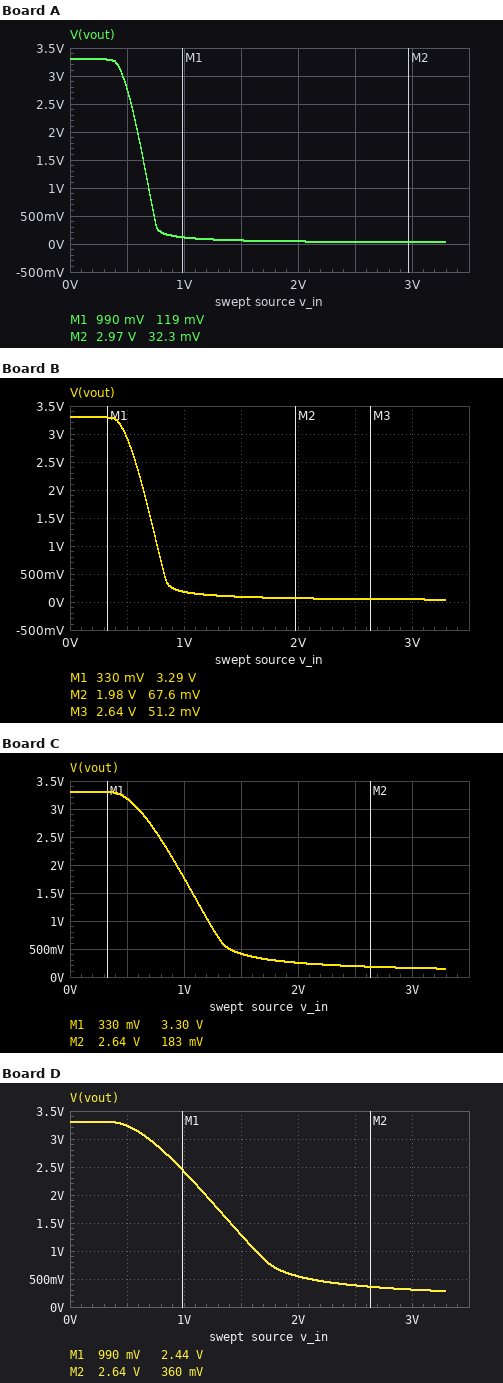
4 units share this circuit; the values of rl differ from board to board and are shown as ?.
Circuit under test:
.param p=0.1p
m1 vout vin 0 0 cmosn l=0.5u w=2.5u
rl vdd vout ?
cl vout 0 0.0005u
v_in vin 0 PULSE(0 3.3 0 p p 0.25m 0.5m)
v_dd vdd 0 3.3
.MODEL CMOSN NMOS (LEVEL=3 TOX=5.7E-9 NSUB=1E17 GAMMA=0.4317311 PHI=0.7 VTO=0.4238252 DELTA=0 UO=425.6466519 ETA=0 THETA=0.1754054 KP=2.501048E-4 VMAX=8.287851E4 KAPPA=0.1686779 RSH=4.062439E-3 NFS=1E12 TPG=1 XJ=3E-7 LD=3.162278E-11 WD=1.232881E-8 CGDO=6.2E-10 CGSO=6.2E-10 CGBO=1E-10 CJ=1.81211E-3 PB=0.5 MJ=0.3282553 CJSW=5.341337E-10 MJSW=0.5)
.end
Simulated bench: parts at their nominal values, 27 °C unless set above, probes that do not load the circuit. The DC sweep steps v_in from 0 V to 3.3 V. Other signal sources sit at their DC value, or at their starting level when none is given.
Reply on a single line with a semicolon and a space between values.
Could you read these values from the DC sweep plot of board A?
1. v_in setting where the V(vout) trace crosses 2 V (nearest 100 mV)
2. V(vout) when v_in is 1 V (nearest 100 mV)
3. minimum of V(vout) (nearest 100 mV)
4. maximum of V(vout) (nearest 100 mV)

600 mV; 100 mV; 0 V; 3.3 V
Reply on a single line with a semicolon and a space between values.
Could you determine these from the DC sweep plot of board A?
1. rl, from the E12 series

47 kΩ
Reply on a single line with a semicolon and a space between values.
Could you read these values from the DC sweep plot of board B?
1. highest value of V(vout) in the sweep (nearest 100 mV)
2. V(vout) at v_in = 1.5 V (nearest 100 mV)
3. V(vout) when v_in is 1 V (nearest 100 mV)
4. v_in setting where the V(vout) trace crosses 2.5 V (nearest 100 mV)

3.3 V; 100 mV; 200 mV; 600 mV
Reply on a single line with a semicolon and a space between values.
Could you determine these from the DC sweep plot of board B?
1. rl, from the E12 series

33 kΩ
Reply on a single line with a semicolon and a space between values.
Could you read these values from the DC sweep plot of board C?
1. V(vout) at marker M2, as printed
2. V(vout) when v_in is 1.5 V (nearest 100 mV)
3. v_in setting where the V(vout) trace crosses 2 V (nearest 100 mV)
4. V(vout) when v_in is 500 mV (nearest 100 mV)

183 mV; 400 mV; 900 mV; 3.2 V
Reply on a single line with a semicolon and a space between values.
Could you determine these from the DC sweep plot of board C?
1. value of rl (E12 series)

10 kΩ
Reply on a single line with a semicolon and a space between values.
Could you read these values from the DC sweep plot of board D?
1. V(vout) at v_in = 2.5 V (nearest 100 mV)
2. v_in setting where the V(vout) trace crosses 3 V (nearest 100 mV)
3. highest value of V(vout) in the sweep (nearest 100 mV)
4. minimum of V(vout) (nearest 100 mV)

400 mV; 700 mV; 3.3 V; 300 mV
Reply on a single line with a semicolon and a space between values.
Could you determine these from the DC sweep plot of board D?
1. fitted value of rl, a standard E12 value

5.6 kΩ
